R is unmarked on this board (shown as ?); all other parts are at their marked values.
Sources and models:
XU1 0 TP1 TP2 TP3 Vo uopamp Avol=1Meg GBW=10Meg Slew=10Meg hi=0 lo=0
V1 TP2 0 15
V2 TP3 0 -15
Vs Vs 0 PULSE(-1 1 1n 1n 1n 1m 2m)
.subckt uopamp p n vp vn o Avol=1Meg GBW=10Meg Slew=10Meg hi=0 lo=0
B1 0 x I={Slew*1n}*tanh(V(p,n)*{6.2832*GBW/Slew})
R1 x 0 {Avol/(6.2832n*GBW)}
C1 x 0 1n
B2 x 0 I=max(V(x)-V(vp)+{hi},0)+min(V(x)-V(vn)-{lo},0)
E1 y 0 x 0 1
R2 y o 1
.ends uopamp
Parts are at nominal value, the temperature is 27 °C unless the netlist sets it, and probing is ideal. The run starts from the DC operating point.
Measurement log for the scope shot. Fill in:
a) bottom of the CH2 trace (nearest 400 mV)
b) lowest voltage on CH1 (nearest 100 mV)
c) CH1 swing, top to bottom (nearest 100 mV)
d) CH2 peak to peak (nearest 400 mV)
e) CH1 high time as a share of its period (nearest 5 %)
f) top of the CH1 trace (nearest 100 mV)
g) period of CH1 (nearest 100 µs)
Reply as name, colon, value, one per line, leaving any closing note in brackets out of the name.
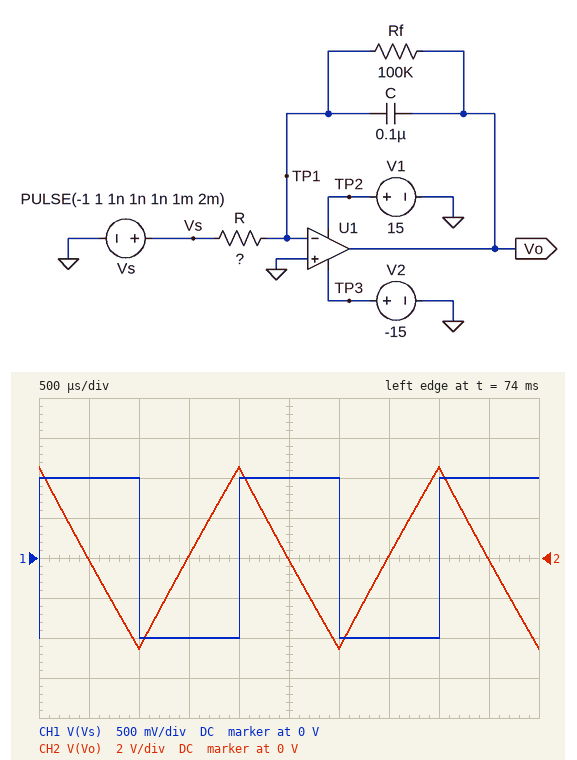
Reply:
bottom of the CH2 trace: -4.4 V
lowest voltage on CH1: -1.0 V
CH1 swing, top to bottom: 2.0 V
CH2 peak to peak: 9.2 V
CH1 high time as a share of its period: 50 %
top of the CH1 trace: 1.0 V
period of CH1: 2.0 ms
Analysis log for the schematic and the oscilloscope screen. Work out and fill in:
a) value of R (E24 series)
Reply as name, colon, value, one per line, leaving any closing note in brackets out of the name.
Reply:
value of R: 1.1 kΩ
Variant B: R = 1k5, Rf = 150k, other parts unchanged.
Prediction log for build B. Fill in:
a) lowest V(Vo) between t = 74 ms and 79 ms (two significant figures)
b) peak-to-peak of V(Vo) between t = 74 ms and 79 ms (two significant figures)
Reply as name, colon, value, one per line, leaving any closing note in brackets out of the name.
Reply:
lowest V(Vo) between t = 74 ms and 79 ms: -3.3 V
peak-to-peak of V(Vo) between t = 74 ms and 79 ms: 6.7 V
